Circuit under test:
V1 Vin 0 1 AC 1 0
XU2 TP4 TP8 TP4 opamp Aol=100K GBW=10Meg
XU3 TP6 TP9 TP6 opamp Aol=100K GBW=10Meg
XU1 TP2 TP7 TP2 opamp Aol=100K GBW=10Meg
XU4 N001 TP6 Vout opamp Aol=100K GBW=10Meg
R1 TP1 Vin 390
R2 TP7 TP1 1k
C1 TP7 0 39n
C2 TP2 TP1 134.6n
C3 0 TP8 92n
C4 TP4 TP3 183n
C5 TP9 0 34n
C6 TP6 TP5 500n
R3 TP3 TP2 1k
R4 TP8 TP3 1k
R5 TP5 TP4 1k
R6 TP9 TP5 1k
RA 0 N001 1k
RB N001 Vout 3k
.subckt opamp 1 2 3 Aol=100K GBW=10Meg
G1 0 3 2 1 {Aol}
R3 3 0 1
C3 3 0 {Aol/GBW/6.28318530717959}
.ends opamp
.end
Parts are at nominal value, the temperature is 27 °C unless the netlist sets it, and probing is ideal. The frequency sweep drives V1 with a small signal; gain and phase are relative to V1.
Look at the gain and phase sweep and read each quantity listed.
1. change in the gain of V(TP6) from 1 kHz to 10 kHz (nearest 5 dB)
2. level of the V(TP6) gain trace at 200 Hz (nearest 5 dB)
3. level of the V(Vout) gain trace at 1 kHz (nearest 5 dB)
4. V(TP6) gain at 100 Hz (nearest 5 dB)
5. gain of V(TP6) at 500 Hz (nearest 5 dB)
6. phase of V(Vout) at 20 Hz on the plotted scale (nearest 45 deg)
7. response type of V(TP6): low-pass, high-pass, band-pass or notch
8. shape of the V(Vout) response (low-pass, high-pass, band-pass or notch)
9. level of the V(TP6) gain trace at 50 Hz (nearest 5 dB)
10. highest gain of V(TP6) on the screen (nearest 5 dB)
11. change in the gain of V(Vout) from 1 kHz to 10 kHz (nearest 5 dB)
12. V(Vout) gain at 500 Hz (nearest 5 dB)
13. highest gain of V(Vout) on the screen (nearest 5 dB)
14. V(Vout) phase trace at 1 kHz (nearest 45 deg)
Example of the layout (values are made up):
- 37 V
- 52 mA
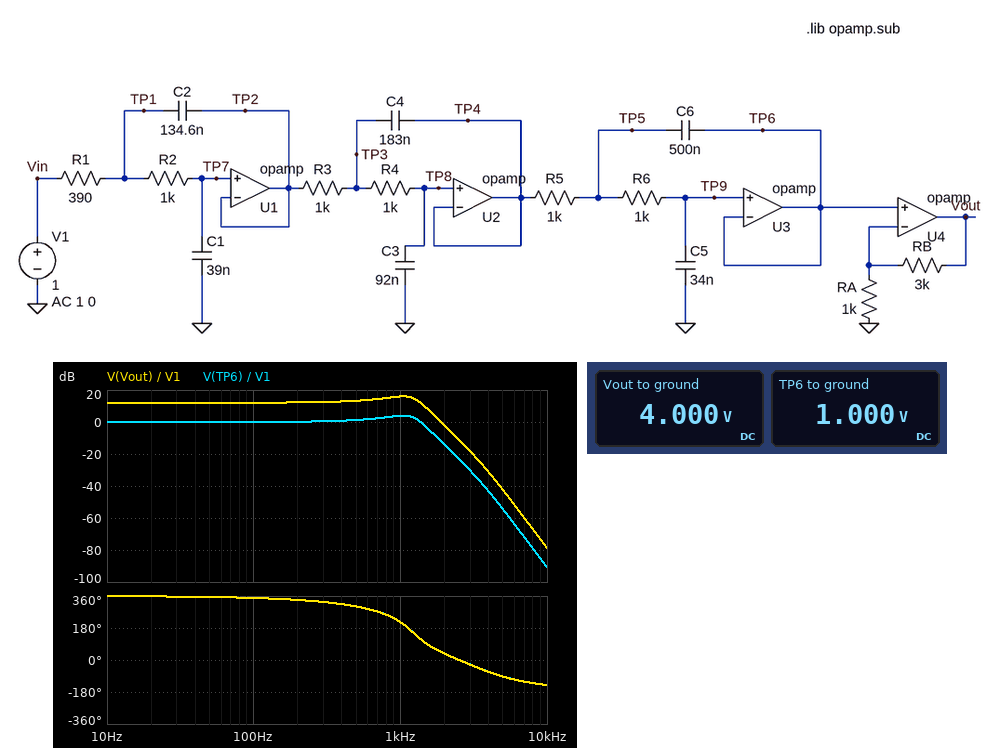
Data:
- -95 dB
- 0 dB
- 15 dB
- 0 dB
- 0 dB
- 360 deg
- low-pass
- low-pass
- 0 dB
- 5 dB
- -95 dB
- 15 dB
- 15 dB
- 225 deg
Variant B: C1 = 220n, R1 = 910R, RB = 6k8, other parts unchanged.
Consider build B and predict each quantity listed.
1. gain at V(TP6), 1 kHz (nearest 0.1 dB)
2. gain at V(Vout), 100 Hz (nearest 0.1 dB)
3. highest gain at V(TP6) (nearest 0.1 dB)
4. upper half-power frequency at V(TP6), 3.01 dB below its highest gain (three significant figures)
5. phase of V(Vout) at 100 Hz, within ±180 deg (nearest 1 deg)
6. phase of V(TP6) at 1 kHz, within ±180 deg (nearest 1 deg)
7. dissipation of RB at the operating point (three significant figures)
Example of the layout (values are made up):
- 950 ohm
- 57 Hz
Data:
- -4.7 dB
- 17.7 dB
- 0 dB
- 617 Hz
- -24 deg
- 142 deg
- 6.80 mW
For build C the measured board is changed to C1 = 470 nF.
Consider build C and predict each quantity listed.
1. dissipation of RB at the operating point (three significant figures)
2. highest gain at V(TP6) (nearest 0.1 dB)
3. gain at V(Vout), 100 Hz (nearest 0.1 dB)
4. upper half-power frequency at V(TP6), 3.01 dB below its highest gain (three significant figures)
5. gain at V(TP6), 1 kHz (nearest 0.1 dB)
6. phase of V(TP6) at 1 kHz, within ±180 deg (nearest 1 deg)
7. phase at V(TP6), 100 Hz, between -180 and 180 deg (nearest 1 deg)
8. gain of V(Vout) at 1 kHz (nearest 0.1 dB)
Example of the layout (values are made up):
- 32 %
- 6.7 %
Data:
- 3.00 mW
- 0 dB
- 11.5 dB
- 282 Hz
- -8.5 dB
- 144 deg
- -32 deg
- 3.5 dB
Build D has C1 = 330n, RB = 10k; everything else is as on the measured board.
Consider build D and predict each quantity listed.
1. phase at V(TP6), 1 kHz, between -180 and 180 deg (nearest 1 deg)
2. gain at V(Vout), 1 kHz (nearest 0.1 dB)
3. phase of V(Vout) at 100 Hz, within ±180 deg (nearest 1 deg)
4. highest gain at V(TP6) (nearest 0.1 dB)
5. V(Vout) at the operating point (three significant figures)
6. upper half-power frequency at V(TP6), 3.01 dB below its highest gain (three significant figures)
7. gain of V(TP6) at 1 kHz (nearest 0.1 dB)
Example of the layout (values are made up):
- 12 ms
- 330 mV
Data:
- 150 deg
- 15.3 dB
- -25 deg
- 0 dB
- 11.0 V
- 469 Hz
- -5.5 dB
